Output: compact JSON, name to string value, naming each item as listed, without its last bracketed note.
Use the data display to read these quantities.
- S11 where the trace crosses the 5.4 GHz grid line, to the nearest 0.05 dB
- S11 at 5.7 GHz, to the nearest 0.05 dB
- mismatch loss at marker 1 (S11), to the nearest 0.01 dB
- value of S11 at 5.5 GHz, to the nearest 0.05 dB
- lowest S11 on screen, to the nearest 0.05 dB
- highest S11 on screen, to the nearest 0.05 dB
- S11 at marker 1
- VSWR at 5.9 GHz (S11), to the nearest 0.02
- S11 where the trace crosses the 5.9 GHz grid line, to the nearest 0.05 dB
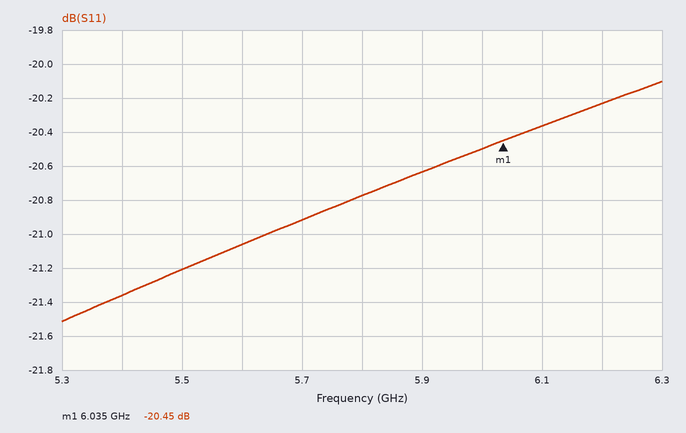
{"S11 where the trace crosses the 5.4 GHz grid line, to the nearest 0.05 dB": "-21.35 dB", "S11 at 5.7 GHz, to the nearest 0.05 dB": "-20.90 dB", "mismatch loss at marker 1 (S11), to the nearest 0.01 dB": "0.04 dB", "value of S11 at 5.5 GHz, to the nearest 0.05 dB": "-21.20 dB", "lowest S11 on screen, to the nearest 0.05 dB": "-21.50 dB", "highest S11 on screen, to the nearest 0.05 dB": "-20.10 dB", "S11 at marker 1": "-20.45 dB", "VSWR at 5.9 GHz (S11), to the nearest 0.02": "1.20", "S11 where the trace crosses the 5.9 GHz grid line, to the nearest 0.05 dB": "-20.65 dB"}
